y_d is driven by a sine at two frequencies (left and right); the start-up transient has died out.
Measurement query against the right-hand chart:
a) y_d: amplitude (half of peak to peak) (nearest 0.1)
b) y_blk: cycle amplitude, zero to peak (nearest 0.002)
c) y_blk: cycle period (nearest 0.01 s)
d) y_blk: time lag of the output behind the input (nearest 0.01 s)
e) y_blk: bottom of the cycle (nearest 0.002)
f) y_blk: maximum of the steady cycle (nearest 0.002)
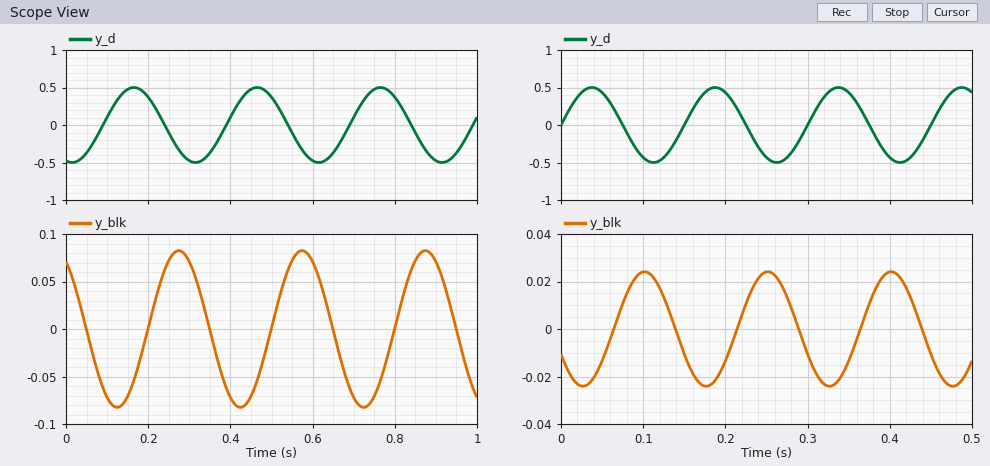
0.5
0.024
0.15 s
0.06 s
-0.024
0.024
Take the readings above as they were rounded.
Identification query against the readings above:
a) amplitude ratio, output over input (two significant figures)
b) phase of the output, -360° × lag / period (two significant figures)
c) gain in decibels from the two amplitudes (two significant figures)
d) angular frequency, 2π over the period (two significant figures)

0.048
-140°
-26 dB
42 rad/s
